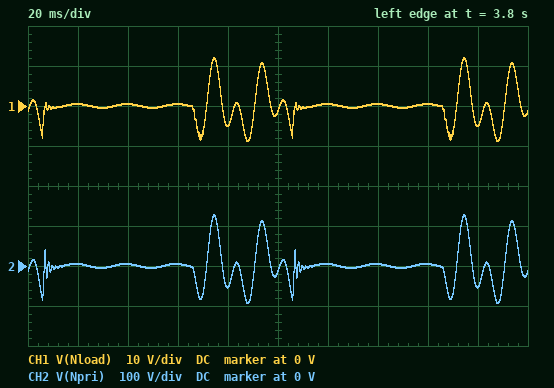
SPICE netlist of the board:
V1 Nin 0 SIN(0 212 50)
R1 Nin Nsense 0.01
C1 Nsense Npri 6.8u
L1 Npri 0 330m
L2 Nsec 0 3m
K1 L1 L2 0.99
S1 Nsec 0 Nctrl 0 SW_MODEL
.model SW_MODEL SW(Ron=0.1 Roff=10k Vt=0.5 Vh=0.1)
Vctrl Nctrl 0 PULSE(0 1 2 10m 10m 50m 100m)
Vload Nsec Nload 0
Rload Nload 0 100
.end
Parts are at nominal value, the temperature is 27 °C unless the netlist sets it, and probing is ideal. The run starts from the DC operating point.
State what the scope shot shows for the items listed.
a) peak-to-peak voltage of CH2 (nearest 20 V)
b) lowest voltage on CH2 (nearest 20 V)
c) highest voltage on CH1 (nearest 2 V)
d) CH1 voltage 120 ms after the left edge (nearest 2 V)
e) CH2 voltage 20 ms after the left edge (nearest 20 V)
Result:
220 V
-100 V
12 V
0 V
0 V
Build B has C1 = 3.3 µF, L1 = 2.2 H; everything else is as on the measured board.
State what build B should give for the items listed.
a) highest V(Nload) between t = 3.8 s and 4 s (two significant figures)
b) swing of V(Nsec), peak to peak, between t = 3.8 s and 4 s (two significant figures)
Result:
31 V
65 V
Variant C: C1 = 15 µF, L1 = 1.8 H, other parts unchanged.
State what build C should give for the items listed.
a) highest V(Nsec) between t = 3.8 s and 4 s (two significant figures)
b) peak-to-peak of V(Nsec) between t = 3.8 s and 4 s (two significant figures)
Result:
25 V
51 V
